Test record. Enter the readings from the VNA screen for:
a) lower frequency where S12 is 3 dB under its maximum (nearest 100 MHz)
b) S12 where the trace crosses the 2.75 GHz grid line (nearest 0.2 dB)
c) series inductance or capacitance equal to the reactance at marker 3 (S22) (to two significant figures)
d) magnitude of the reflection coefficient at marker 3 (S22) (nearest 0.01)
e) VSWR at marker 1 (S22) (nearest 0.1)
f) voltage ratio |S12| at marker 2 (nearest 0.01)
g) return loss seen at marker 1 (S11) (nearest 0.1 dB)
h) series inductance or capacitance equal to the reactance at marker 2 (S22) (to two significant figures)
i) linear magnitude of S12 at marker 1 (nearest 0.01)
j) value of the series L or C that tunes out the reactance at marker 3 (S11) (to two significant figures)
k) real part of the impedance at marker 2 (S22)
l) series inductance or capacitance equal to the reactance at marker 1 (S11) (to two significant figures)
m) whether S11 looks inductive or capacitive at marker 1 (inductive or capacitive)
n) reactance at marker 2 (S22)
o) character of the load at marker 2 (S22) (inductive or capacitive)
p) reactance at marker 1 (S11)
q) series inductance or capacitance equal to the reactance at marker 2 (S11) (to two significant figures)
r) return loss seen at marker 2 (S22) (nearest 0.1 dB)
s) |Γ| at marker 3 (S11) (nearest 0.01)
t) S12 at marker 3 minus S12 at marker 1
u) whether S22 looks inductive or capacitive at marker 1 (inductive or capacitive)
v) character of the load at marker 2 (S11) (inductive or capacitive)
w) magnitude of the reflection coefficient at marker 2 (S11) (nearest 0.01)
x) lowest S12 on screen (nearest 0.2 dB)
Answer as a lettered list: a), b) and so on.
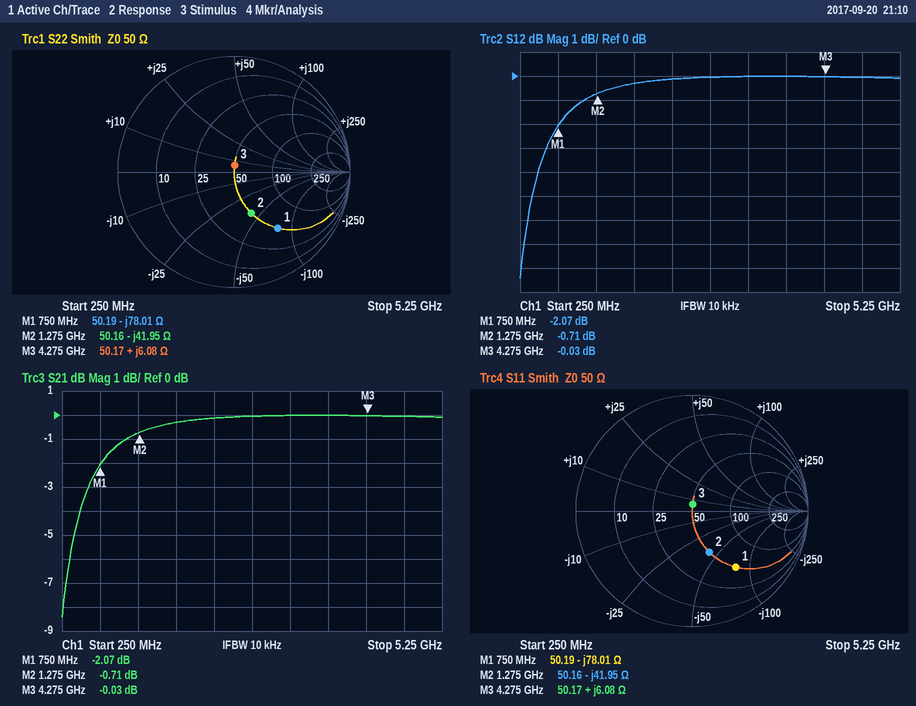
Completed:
a) 600 MHz
b) 0.0 dB
c) 230 pH
d) 0.06
e) 4.2
f) 0.92
g) 4.2 dB
h) 3.0 pF
i) 0.79
j) 6.1 pF
k) 50.16 Ω
l) 2.7 pF
m) capacitive
n) -41.95 Ω
o) capacitive
p) -78.01 Ω
q) 3.0 pF
r) 8.3 dB
s) 0.06
t) 2.04 dB
u) capacitive
v) capacitive
w) 0.39
x) -8.4 dB
